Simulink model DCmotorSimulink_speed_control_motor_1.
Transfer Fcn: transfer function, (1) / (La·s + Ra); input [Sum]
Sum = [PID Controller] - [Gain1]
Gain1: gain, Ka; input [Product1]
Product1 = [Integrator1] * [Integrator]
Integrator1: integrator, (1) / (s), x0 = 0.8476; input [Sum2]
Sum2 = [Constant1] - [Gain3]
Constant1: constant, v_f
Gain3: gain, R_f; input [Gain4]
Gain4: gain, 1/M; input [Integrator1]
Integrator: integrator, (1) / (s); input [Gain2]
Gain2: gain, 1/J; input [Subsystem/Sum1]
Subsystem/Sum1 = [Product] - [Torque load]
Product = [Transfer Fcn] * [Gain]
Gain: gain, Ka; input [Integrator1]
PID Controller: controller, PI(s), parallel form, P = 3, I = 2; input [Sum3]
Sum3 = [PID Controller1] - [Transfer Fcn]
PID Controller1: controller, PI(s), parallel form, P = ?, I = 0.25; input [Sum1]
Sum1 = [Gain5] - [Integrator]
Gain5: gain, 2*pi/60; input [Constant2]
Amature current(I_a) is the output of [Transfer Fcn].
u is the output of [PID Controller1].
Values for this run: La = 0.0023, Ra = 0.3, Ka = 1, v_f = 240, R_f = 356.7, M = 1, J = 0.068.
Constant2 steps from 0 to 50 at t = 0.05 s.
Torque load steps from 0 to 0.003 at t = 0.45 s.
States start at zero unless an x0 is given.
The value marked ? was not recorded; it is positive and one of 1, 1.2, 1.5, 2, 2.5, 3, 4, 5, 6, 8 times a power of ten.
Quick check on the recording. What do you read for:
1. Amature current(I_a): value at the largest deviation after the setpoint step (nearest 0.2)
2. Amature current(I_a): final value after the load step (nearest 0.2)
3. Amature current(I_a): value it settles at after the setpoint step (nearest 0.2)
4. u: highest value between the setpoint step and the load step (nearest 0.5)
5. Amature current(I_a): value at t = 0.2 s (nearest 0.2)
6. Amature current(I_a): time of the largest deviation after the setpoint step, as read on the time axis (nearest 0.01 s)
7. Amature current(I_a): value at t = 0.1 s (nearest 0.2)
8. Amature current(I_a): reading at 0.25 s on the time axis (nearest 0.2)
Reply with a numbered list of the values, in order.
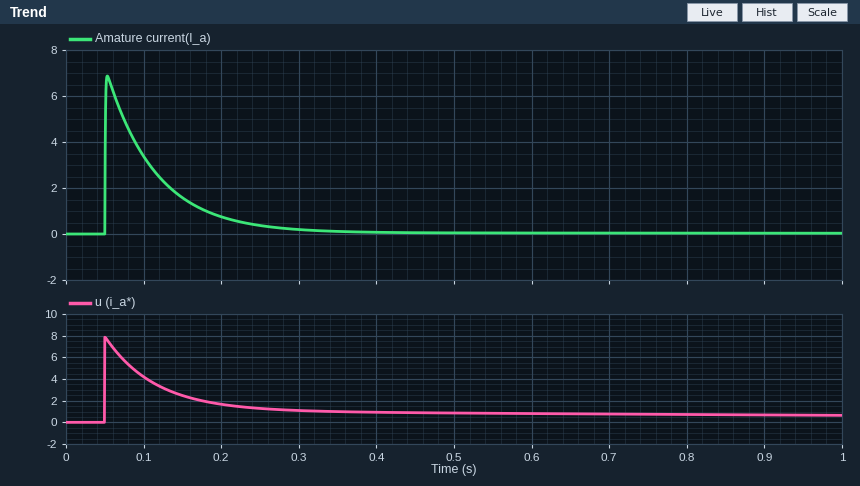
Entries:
1. 6.8
2. 0.0
3. 0.0
4. 8.0
5. 0.8
6. 0.05 s
7. 3.4
8. 0.4
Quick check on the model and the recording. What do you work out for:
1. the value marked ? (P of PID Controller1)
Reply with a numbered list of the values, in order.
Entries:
1. 1.5
